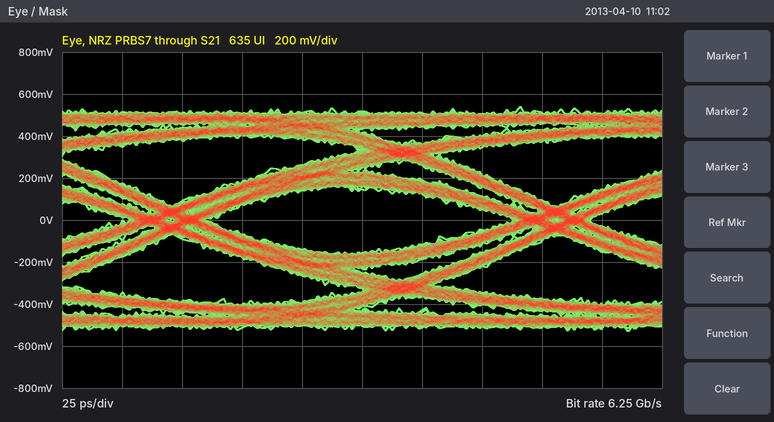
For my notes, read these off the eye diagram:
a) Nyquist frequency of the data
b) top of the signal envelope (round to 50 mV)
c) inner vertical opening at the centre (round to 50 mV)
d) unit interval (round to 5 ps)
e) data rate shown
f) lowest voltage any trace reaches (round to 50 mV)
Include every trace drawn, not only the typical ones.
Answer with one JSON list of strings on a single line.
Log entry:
["3.125 GHz", "550 mV", "300 mV", "160 ps", "6.25 Gb/s", "-550 mV"]
